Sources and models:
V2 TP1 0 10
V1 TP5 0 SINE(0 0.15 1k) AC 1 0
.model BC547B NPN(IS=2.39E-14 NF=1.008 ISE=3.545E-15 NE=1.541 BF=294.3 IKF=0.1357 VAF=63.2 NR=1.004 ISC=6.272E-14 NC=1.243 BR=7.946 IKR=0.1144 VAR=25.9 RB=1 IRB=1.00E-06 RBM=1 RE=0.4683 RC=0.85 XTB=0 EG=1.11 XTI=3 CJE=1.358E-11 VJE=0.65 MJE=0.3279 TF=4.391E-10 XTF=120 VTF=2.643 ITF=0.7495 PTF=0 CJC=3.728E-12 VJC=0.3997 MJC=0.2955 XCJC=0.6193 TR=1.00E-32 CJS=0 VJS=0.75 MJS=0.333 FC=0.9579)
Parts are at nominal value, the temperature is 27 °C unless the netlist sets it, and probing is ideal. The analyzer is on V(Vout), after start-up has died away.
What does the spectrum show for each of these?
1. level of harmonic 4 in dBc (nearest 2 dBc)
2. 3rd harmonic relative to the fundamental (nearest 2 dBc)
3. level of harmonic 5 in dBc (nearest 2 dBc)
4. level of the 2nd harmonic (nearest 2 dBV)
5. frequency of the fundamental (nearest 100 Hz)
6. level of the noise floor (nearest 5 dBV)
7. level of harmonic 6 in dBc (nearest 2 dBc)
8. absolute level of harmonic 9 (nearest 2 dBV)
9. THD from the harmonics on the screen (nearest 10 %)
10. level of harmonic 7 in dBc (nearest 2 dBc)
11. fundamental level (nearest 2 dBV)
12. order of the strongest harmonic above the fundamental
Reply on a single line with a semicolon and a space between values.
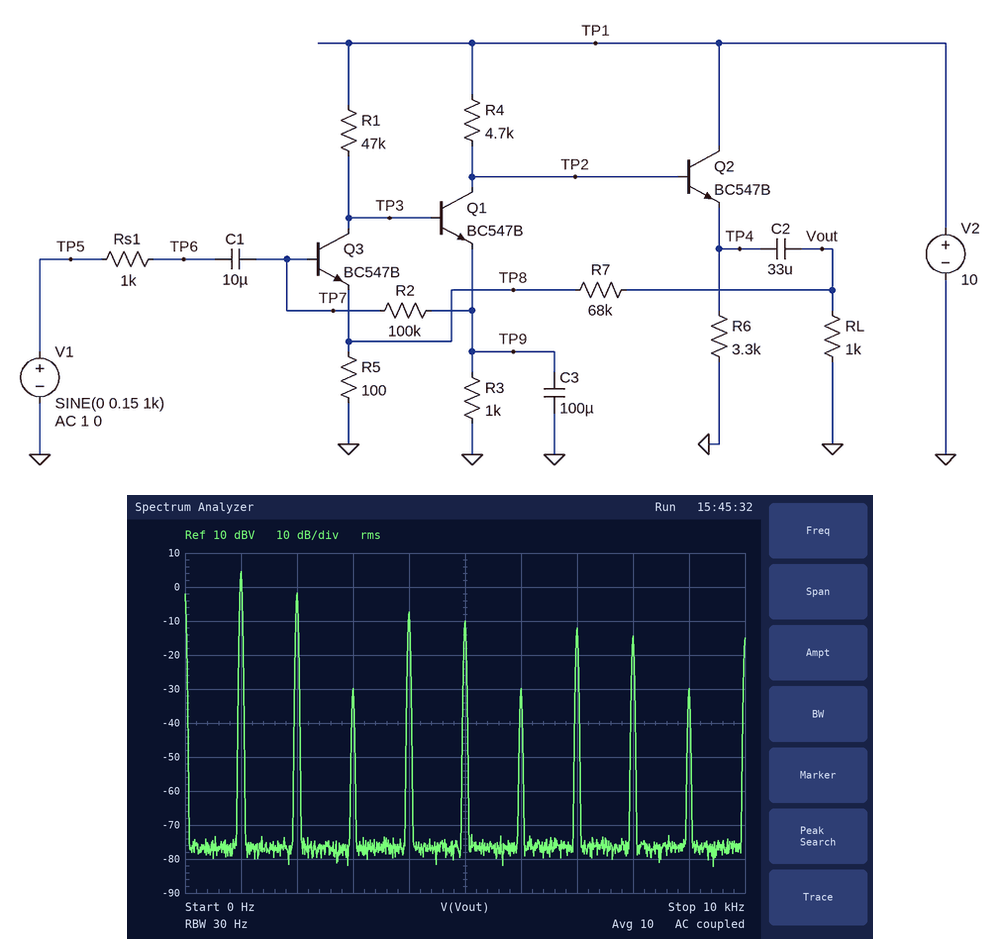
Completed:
-12 dBc; -34 dBc; -14 dBc; -2 dBV; 1.0 kHz; -75 dBV; -34 dBc; -30 dBV; 60 %; -16 dBc; 4 dBV; 2
